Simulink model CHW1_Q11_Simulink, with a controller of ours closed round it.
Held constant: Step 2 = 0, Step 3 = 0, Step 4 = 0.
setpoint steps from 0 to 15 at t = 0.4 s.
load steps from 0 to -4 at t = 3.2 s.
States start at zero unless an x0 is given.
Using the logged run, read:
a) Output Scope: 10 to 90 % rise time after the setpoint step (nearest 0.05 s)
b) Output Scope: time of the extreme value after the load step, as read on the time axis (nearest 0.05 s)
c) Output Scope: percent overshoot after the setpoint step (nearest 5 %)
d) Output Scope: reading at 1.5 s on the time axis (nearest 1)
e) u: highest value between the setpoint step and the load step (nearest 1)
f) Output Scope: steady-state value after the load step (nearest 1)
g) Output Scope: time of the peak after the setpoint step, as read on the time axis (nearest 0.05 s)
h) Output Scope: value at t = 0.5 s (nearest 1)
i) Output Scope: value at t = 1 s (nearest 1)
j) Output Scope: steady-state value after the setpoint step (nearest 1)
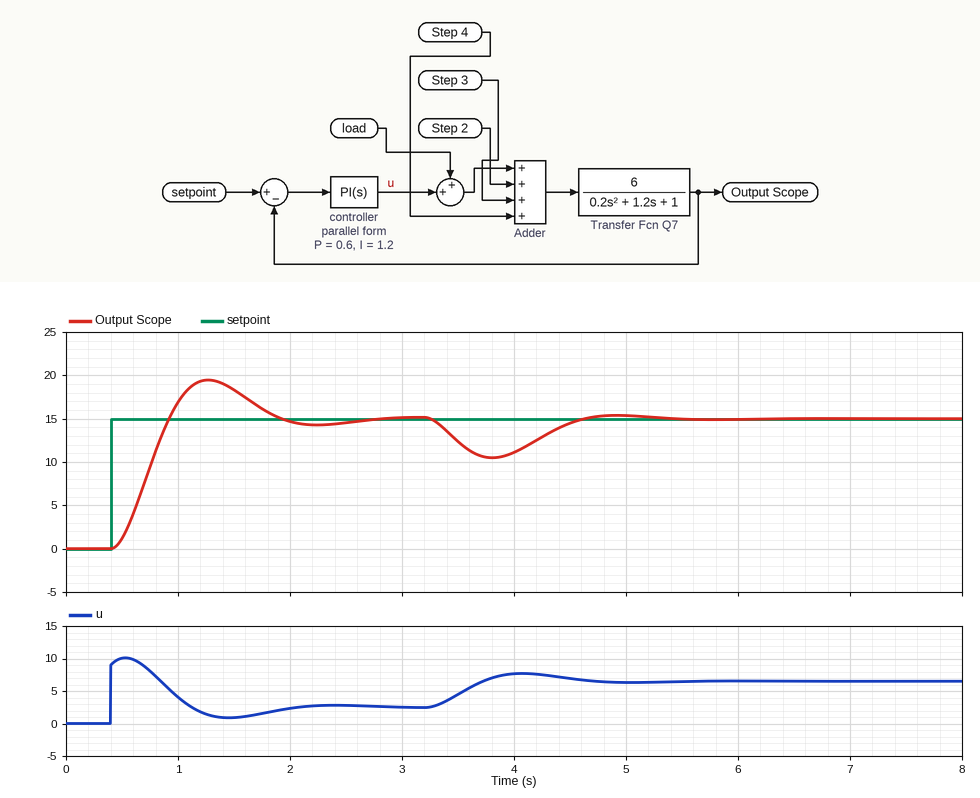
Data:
0.35 s
3.80 s
30 %
18
10
15
1.25 s
1
17
15
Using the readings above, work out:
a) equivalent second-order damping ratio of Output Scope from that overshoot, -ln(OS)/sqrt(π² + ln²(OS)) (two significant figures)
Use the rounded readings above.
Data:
0.36
